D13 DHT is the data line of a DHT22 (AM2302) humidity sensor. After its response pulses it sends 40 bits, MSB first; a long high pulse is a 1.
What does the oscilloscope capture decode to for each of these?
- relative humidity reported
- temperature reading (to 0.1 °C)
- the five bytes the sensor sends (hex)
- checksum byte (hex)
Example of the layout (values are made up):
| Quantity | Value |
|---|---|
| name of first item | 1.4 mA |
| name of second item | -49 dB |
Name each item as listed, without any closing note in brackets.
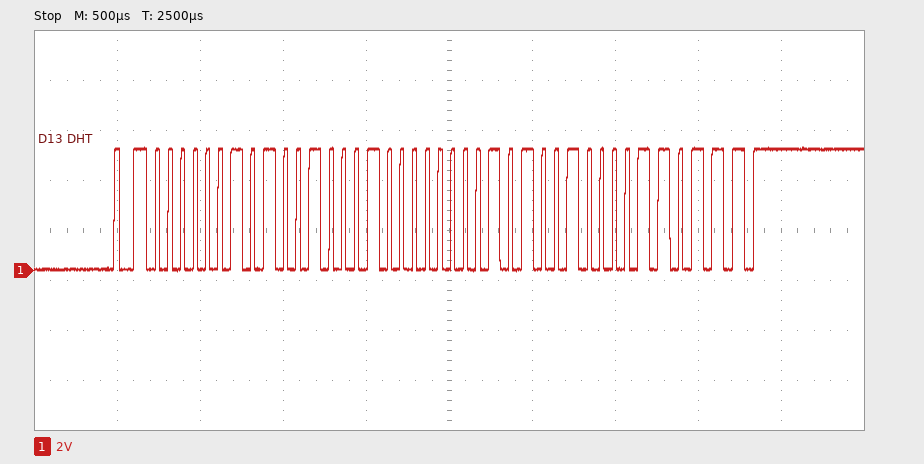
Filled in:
| Quantity | Value |
|---|---|
| relative humidity reported | 65.7 % |
| temperature reading | 16.4 °C |
| the five bytes the sensor sends | 02 91 00 A4 37 |
| checksum byte | 0x37 |
